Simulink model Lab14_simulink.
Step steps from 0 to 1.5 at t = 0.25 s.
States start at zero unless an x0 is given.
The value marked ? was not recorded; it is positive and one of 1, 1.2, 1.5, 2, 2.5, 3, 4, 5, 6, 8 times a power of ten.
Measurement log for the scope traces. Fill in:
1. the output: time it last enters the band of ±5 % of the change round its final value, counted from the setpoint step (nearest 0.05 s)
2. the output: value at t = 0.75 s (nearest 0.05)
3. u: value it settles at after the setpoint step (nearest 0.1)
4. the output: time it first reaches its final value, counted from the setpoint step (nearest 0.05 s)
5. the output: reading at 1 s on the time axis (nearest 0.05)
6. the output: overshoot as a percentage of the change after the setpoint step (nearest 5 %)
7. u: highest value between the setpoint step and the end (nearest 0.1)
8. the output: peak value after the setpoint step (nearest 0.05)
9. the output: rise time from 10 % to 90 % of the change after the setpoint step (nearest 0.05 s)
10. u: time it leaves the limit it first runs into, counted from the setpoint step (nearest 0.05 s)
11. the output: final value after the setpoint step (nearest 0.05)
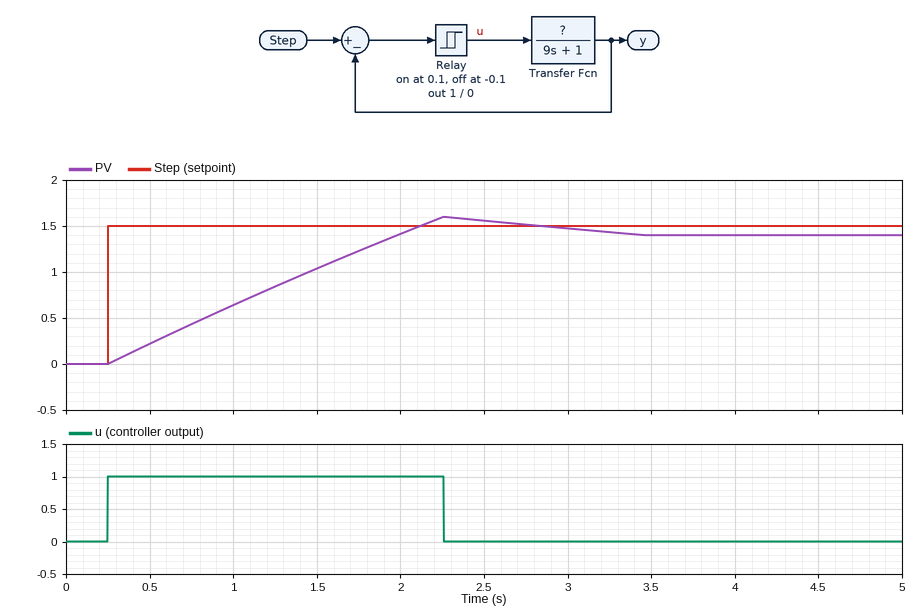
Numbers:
2.75 s
0.45
0.0
1.75 s
0.65
15 %
1.0
1.60
1.40 s
2.00 s
1.40
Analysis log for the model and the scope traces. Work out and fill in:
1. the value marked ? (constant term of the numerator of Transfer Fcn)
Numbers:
8
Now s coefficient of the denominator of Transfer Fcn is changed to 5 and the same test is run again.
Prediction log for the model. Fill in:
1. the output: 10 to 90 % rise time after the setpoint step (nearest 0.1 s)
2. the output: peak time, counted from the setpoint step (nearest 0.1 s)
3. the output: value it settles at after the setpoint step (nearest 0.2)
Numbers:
0.8 s
1.1 s
1.4
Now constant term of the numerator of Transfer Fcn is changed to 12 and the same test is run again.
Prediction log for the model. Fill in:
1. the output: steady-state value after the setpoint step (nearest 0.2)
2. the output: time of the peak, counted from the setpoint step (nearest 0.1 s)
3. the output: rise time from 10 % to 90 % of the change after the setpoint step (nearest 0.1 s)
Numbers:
1.4
1.3 s
0.9 s
